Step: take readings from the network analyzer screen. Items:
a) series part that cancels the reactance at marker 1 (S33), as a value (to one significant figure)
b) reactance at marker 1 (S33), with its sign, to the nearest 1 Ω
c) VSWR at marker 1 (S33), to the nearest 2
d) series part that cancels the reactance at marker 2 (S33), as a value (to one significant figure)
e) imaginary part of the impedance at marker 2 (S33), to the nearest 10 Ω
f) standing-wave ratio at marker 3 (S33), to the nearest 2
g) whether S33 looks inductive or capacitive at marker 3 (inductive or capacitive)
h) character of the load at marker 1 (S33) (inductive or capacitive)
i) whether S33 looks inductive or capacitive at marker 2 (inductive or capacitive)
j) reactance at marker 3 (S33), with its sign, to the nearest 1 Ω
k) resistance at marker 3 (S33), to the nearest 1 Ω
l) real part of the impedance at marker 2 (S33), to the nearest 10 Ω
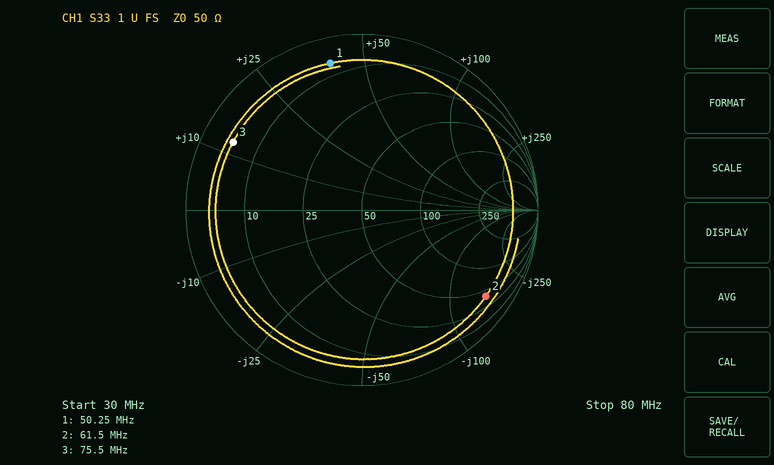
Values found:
80 pF
+40 Ω
12
400 nH
-150 Ω
10
inductive
inductive
capacitive
+12 Ω
5 Ω
40 Ω
